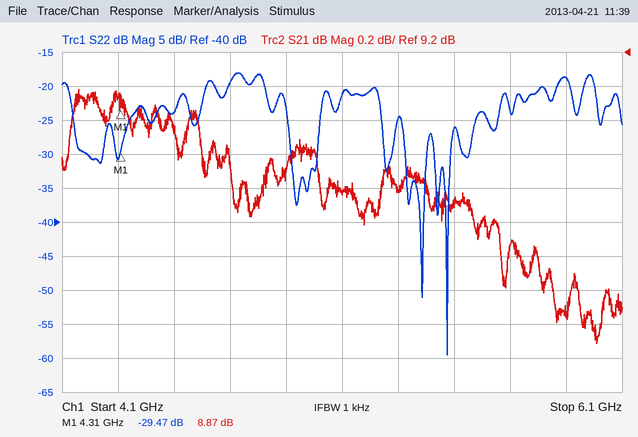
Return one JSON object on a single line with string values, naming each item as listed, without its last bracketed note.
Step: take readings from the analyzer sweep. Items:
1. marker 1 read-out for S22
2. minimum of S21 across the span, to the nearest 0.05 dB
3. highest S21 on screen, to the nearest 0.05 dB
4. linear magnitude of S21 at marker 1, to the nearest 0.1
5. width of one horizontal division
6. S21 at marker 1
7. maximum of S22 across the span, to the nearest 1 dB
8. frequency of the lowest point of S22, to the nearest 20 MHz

{"marker 1 read-out for S22": "-29.47 dB", "minimum of S21 across the span, to the nearest 0.05 dB": "7.50 dB", "highest S21 on screen, to the nearest 0.05 dB": "9.00 dB", "linear magnitude of S21 at marker 1, to the nearest 0.1": "2.8", "width of one horizontal division": "200 MHz", "S21 at marker 1": "8.87 dB", "maximum of S22 across the span, to the nearest 1 dB": "-18 dB", "frequency of the lowest point of S22, to the nearest 20 MHz": "5.48 GHz"}
